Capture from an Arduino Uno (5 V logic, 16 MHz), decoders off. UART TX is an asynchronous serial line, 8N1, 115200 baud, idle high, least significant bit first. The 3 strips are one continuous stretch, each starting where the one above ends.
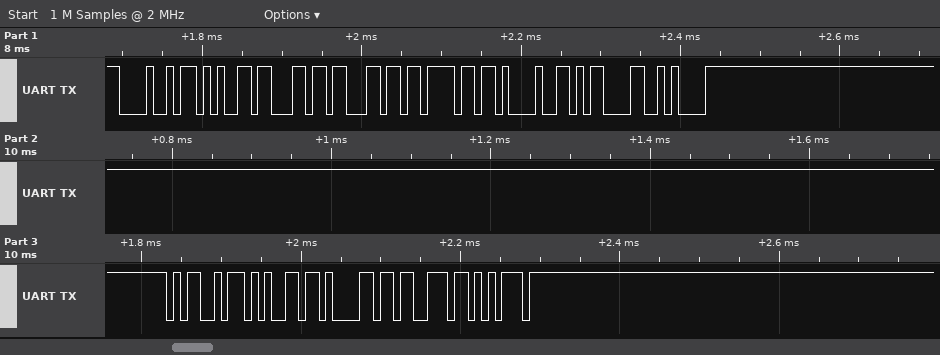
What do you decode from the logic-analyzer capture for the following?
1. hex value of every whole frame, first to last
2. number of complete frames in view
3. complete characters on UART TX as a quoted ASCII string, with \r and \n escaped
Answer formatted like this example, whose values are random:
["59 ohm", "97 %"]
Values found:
["0x48 0x65 0x6C 0x6C 0x6F 0x21 0x0D 0x0A 0x4D 0x65 0x61 0x73 0x75", "13", "\"Hello!\\r\\nMeasu\""]
